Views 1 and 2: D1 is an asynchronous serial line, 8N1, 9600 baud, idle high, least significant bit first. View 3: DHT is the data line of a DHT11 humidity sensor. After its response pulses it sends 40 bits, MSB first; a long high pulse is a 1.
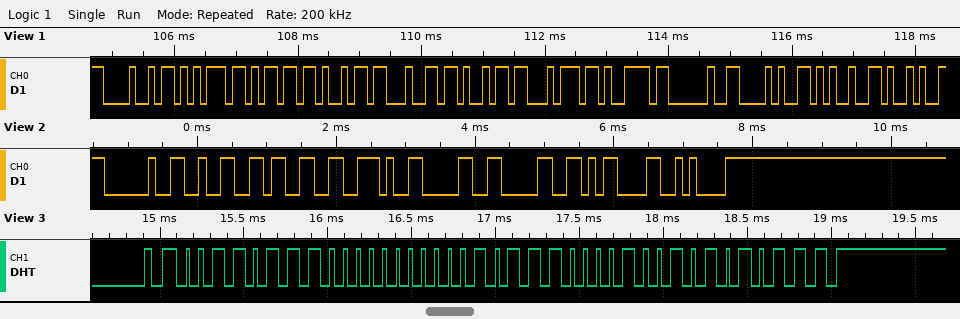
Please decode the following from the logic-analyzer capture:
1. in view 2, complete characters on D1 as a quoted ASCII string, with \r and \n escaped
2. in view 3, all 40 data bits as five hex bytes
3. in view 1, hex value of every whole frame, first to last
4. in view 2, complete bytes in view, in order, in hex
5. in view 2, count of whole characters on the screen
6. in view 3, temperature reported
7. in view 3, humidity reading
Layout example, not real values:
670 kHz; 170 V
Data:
" 23.00\r\n"; 37 00 17 09 57; 0x48 0x75 0x6D 0x69 0x64 0x69 0x74 0x79 0x20 0x28 0x25 0x29; 20 32 33 2E 30 30 0D 0A; 8; 23.9 °C; 55 %
